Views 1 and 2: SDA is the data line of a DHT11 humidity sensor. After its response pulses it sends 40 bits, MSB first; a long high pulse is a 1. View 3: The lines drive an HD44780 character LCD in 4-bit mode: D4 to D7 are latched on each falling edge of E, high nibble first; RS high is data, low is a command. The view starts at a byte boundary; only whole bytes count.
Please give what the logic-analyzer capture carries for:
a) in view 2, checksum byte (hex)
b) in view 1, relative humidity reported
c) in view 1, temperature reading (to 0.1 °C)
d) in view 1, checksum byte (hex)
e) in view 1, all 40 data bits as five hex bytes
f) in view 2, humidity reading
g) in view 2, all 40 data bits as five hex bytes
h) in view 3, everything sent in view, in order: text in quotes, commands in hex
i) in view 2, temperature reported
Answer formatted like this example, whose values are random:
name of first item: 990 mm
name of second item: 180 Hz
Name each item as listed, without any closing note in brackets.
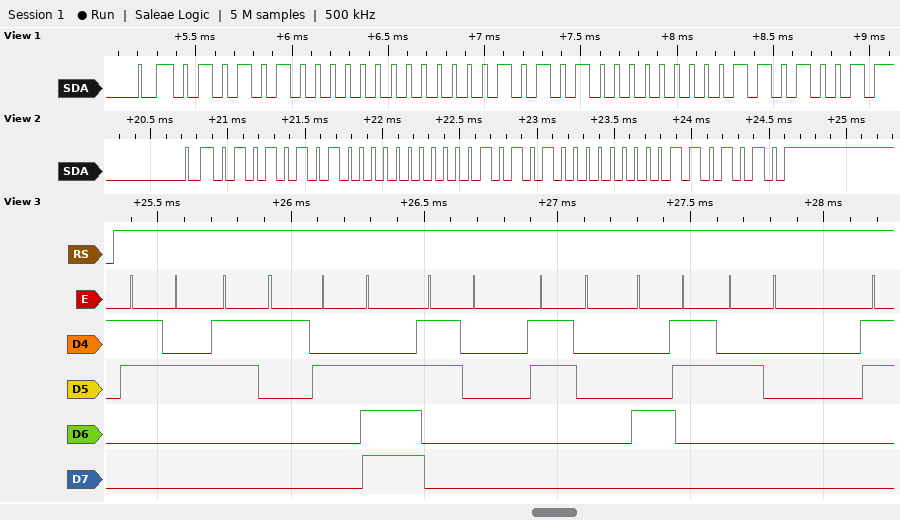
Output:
in view 2, checksum byte: 0x6A
in view 1, relative humidity reported: 84 %
in view 1, temperature reading: 21.0 °C
in view 1, checksum byte: 0x69
in view 1, all 40 data bits as five hex bytes: 54 00 15 00 69
in view 2, humidity reading: 85 %
in view 2, all 40 data bits as five hex bytes: 55 00 15 00 6A
in view 3, everything sent in view, in order: text in quotes, commands in hex: "21.00C "
in view 2, temperature reported: 21.0 °C
